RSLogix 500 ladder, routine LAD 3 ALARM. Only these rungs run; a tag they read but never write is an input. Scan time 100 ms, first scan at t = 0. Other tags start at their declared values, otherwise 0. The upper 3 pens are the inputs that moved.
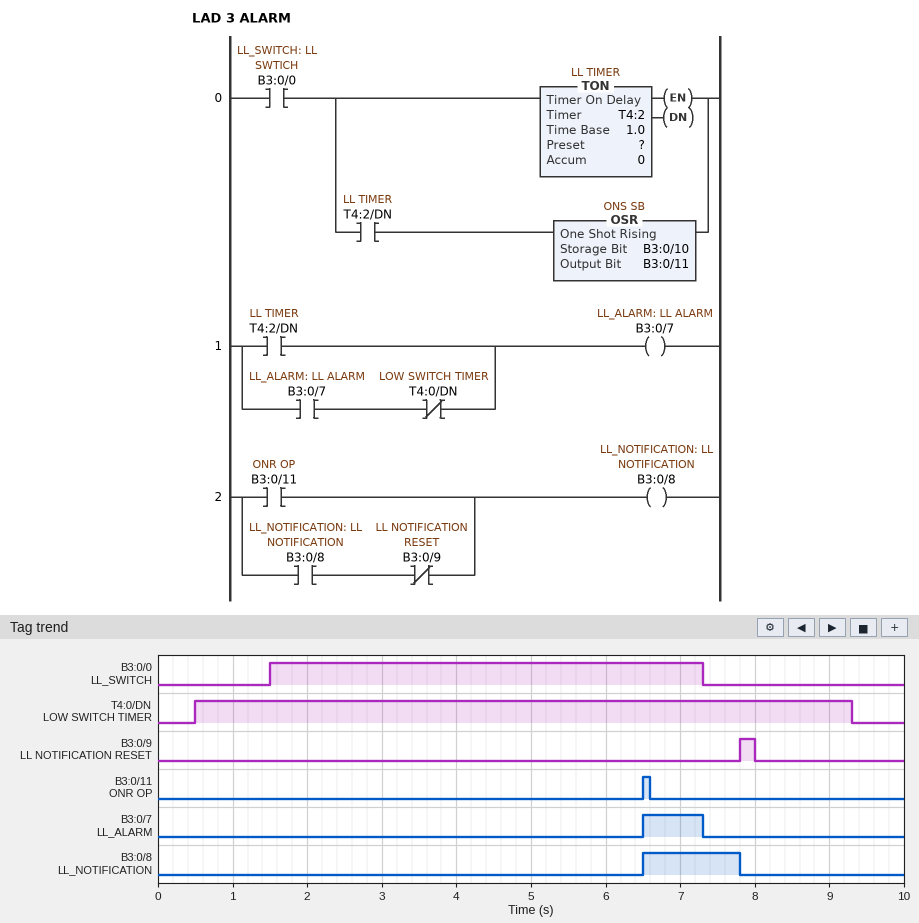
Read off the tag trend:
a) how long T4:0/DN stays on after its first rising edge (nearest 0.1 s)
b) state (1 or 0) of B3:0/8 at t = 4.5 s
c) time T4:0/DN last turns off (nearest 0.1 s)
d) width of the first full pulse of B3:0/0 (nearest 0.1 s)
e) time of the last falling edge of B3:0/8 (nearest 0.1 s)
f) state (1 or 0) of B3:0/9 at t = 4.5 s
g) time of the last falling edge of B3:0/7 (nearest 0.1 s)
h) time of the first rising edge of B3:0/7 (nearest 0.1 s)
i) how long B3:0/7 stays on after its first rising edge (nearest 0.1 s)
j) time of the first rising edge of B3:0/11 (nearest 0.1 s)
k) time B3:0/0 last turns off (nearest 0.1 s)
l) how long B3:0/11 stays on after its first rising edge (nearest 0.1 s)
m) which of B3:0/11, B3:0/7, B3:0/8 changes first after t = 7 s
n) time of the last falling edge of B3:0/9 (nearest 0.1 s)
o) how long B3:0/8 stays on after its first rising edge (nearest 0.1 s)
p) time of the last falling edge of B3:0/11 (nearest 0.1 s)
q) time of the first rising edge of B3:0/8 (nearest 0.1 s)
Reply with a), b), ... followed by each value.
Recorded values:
a) 8.8 s
b) 0
c) 9.3 s
d) 5.8 s
e) 7.8 s
f) 0
g) 7.3 s
h) 6.5 s
i) 0.8 s
j) 6.5 s
k) 7.3 s
l) 0.1 s
m) B3:0/7
n) 8.0 s
o) 1.3 s
p) 6.6 s
q) 6.5 s
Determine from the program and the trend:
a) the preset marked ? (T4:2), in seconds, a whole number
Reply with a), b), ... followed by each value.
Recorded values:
a) 5 s
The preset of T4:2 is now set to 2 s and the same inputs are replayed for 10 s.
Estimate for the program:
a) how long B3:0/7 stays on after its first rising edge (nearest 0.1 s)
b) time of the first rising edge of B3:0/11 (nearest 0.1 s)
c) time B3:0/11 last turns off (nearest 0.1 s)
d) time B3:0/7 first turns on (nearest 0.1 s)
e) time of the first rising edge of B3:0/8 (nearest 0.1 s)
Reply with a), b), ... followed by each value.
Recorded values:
a) 3.8 s
b) 3.5 s
c) 3.6 s
d) 3.5 s
e) 3.5 s
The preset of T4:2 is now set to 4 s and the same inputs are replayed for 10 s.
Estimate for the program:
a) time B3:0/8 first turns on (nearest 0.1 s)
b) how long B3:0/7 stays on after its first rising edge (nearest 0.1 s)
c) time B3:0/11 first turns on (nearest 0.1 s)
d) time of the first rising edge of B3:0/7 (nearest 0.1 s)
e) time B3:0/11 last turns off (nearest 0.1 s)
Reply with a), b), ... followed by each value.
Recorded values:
a) 5.5 s
b) 1.8 s
c) 5.5 s
d) 5.5 s
e) 5.6 s
